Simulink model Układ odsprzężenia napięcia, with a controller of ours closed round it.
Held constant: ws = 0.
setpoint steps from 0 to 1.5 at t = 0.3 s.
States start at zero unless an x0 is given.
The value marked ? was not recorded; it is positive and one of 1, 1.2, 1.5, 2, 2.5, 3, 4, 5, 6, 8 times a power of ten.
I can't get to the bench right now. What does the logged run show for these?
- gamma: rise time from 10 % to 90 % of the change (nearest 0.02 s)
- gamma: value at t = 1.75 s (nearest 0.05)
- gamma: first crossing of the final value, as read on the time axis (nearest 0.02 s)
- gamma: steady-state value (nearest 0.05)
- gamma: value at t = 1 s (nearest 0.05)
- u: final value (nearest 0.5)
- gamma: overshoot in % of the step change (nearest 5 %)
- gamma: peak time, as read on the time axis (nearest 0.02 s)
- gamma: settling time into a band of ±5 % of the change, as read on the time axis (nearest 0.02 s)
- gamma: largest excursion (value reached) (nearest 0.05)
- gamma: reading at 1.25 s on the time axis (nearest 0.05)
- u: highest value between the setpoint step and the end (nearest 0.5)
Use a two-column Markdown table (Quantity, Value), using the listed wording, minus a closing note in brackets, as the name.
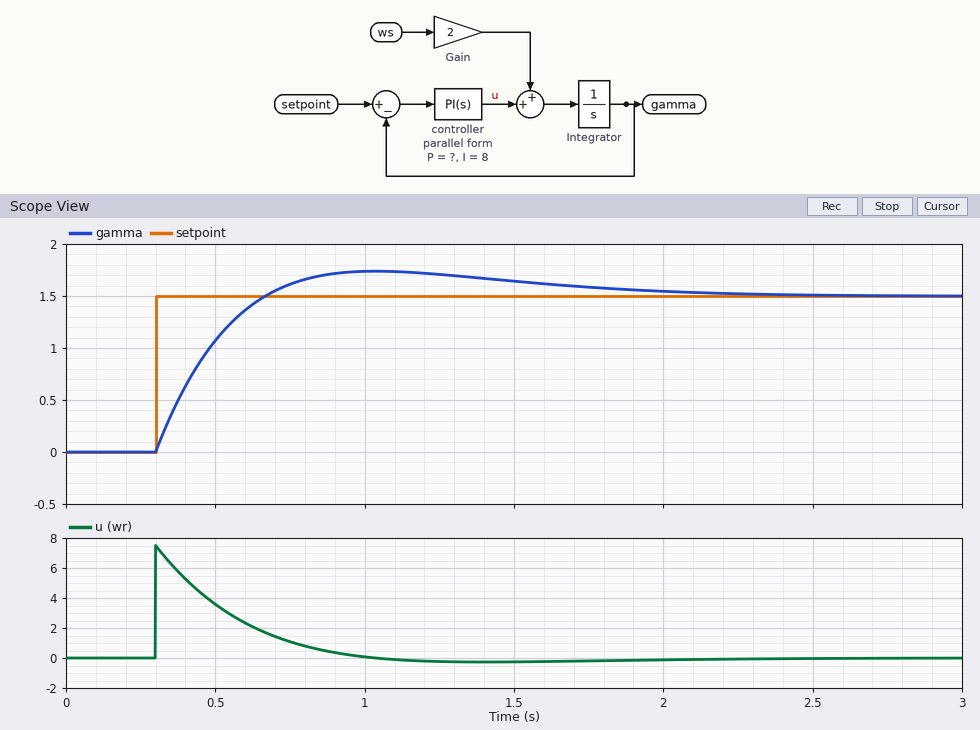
| Quantity | Value |
|---|---|
| gamma: rise time from 10 % to 90 % of the change | 0.28 s |
| gamma: value at t = 1.75 s | 1.60 |
| gamma: first crossing of the final value, as read on the time axis | 0.66 s |
| gamma: steady-state value | 1.50 |
| gamma: value at t = 1 s | 1.75 |
| u: final value | 0.0 |
| gamma: overshoot in % of the step change | 15 % |
| gamma: peak time, as read on the time axis | 1.04 s |
| gamma: settling time into a band of ±5 % of the change, as read on the time axis | 1.80 s |
| gamma: largest excursion (value reached) | 1.75 |
| gamma: reading at 1.25 s on the time axis | 1.70 |
| u: highest value between the setpoint step and the end | 7.5 |
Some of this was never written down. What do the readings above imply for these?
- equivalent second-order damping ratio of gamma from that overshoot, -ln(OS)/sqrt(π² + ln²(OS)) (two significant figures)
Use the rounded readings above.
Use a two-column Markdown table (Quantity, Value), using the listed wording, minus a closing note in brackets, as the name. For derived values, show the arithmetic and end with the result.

| Quantity | Value |
|---|---|
| equivalent second-order damping ratio of gamma from that overshoot, -ln(OS)/sqrt(π² + ln²(OS)) | ln(0.15) = -1.897; 1.897 / sqrt(9.870 + 3.599) = 0.52 |
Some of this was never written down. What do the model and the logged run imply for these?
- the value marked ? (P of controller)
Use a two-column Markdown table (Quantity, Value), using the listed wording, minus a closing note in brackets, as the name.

| Quantity | Value |
|---|---|
| the value marked ? | 5 |
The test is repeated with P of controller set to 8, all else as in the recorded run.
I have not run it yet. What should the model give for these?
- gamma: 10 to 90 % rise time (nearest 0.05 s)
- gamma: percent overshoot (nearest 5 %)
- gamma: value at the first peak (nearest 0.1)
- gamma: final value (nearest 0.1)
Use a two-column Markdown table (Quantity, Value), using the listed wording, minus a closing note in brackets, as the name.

| Quantity | Value |
|---|---|
| gamma: 10 to 90 % rise time | 0.20 s |
| gamma: percent overshoot | 10 % |
| gamma: value at the first peak | 1.6 |
| gamma: final value | 1.5 |
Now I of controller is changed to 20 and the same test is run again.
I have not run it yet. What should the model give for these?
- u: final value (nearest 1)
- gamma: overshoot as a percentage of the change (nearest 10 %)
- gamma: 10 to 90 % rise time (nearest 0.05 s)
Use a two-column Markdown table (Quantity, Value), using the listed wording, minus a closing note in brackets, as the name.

| Quantity | Value |
|---|---|
| u: final value | 0 |
| gamma: overshoot as a percentage of the change | 30 % |
| gamma: 10 to 90 % rise time | 0.20 s |
